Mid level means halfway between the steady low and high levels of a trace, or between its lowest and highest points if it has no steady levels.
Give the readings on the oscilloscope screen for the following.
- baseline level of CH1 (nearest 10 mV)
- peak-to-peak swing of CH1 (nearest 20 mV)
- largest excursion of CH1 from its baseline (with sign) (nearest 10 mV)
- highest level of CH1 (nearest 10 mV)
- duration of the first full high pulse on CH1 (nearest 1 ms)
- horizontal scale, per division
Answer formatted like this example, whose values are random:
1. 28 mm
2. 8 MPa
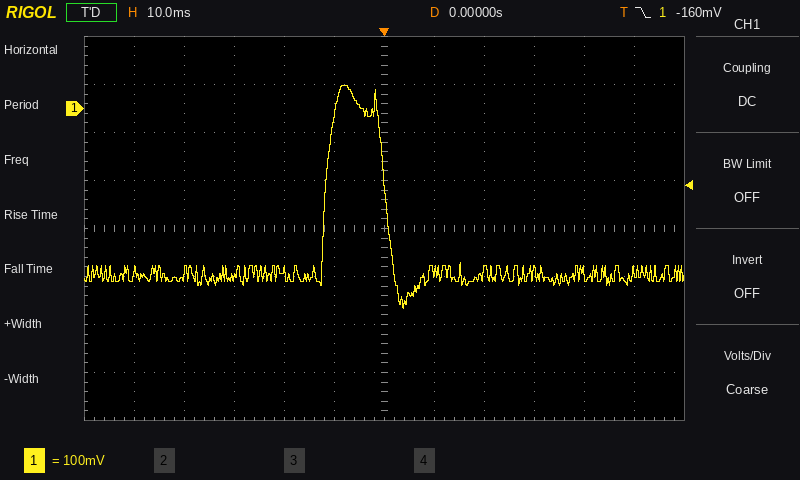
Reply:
1. -350 mV
2. 460 mV
3. +400 mV
4. 50 mV
5. 12 ms
6. 10 ms
